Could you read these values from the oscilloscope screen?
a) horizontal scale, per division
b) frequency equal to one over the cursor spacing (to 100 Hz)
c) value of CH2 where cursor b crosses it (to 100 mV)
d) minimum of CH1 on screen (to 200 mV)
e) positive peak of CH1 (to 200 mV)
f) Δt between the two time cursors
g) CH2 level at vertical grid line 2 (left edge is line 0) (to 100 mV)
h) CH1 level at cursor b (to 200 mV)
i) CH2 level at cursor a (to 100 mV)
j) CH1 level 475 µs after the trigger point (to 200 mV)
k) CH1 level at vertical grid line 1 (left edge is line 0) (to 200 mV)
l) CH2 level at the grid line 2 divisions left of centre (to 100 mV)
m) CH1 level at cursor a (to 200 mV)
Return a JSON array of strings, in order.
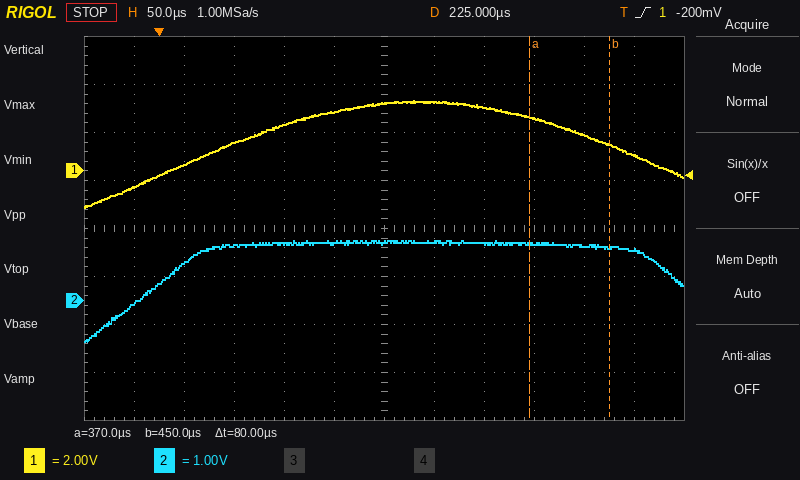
["50 µs", "12.5 kHz", "1.1 V", "-1.6 V", "3.0 V", "80 µs", "800 mV", "1.0 V", "1.2 V", "600 mV", "-600 mV", "1.2 V", "2.2 V"]
